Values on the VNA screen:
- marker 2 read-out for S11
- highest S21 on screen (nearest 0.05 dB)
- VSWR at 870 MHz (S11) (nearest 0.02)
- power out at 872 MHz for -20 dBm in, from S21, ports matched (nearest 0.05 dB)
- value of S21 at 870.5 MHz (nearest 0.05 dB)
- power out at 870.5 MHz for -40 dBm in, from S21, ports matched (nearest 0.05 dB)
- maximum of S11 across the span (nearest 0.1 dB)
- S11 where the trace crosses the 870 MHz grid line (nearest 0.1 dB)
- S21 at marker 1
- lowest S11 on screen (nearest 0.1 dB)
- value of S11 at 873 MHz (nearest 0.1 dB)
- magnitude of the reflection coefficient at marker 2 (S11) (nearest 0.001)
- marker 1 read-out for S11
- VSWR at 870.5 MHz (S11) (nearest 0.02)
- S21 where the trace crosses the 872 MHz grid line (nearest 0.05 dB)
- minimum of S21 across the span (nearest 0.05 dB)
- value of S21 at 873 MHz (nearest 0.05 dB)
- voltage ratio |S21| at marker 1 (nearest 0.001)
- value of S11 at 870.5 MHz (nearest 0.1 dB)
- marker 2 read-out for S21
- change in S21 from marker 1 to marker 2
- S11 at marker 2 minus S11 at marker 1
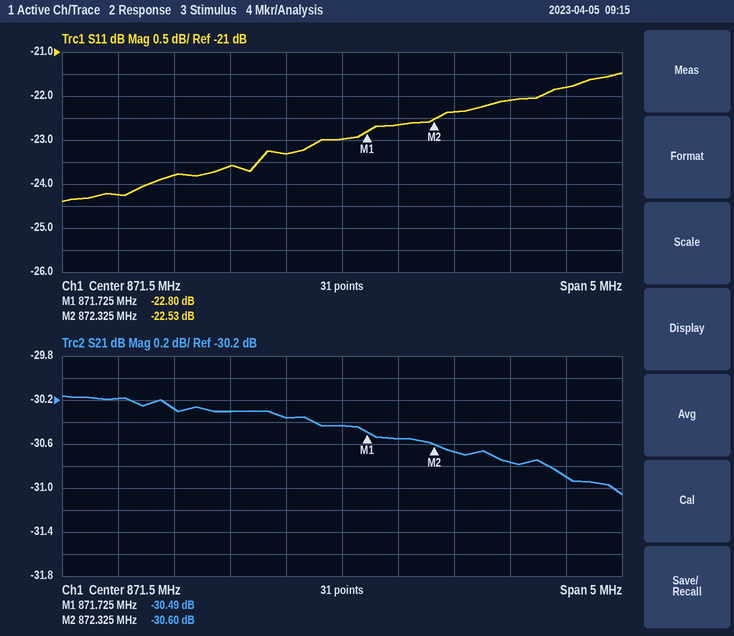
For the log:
-22.53 dB
-30.15 dB
1.14
-50.55 dBm
-30.30 dB
-70.30 dBm
-21.5 dB
-23.8 dB
-30.49 dB
-24.4 dB
-22.1 dB
0.075
-22.80 dB
1.14
-30.55 dB
-31.05 dB
-30.75 dB
0.030
-23.6 dB
-30.60 dB
-0.11 dB
0.27 dB
